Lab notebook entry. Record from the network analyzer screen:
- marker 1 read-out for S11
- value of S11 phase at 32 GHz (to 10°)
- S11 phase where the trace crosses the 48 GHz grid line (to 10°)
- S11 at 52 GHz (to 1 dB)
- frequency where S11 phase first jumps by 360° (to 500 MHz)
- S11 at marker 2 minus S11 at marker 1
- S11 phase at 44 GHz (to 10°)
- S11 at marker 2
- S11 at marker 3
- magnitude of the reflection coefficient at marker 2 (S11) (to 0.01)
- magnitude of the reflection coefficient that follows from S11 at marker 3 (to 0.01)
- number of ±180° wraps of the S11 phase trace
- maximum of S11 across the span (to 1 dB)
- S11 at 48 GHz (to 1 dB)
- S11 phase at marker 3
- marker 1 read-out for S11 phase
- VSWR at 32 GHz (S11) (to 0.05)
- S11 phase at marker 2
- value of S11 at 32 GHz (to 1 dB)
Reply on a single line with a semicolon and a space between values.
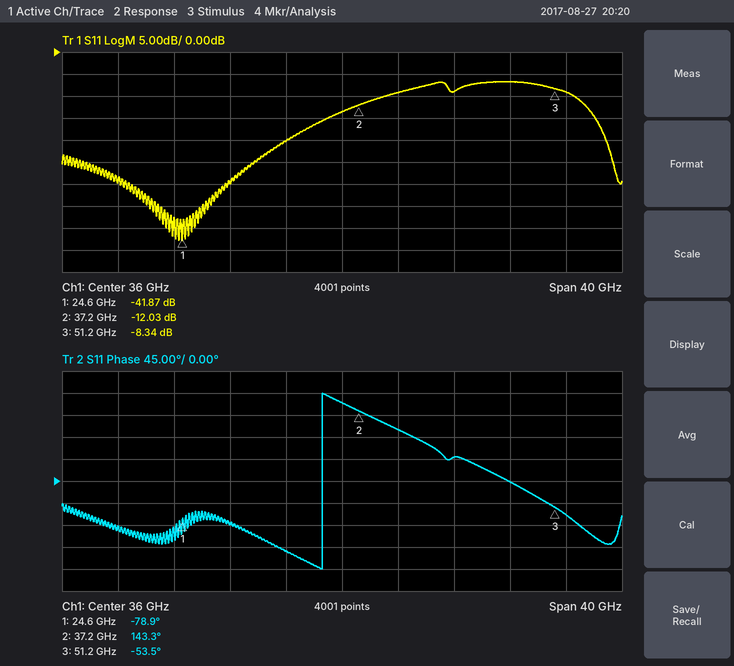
-41.87 dB; -140°; 0°; -9 dB; 34.5 GHz; 29.84 dB; 50°; -12.03 dB; -8.34 dB; 0.25; 0.38; 1; -7 dB; -7 dB; -53.5°; -78.9°; 1.20; 143.3°; -20 dB
